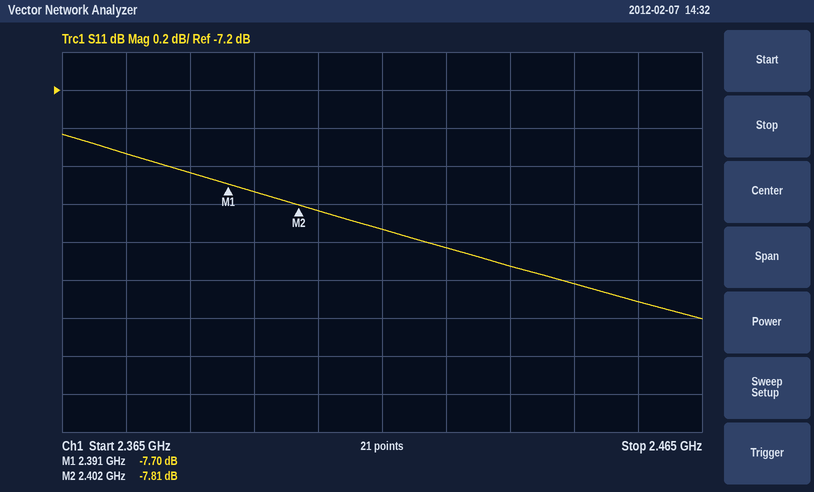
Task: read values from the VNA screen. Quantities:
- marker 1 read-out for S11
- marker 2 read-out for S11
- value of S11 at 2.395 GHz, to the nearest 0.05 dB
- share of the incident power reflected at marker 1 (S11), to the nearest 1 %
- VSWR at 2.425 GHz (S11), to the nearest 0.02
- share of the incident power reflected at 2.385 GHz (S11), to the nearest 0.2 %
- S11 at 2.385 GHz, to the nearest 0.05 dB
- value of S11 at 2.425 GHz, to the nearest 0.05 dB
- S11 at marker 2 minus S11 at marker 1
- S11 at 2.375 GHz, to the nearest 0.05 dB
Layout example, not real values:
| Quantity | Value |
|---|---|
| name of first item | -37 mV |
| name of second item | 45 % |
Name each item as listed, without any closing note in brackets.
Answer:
| Quantity | Value |
|---|---|
| marker 1 read-out for S11 | -7.70 dB |
| marker 2 read-out for S11 | -7.81 dB |
| value of S11 at 2.395 GHz, to the nearest 0.05 dB | -7.75 dB |
| share of the incident power reflected at marker 1 (S11), to the nearest 1 % | 17 % |
| VSWR at 2.425 GHz (S11), to the nearest 0.02 | 2.32 |
| share of the incident power reflected at 2.385 GHz (S11), to the nearest 0.2 % | 17.2 % |
| S11 at 2.385 GHz, to the nearest 0.05 dB | -7.65 dB |
| value of S11 at 2.425 GHz, to the nearest 0.05 dB | -8.05 dB |
| S11 at marker 2 minus S11 at marker 1 | -0.11 dB |
| S11 at 2.375 GHz, to the nearest 0.05 dB | -7.55 dB |
